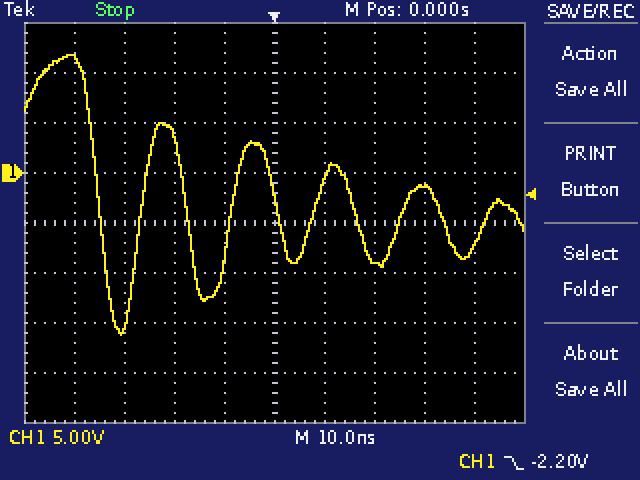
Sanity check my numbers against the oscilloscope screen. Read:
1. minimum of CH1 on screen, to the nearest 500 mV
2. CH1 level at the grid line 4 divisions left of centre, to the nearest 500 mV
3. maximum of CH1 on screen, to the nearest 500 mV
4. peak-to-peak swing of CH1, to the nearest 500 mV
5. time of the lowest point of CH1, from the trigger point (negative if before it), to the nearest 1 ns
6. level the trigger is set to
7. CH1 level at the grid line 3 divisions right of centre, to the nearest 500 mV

-16.0 V
11.5 V
12.0 V
28.0 V
-31 ns
-2.20 V
-1.5 V
